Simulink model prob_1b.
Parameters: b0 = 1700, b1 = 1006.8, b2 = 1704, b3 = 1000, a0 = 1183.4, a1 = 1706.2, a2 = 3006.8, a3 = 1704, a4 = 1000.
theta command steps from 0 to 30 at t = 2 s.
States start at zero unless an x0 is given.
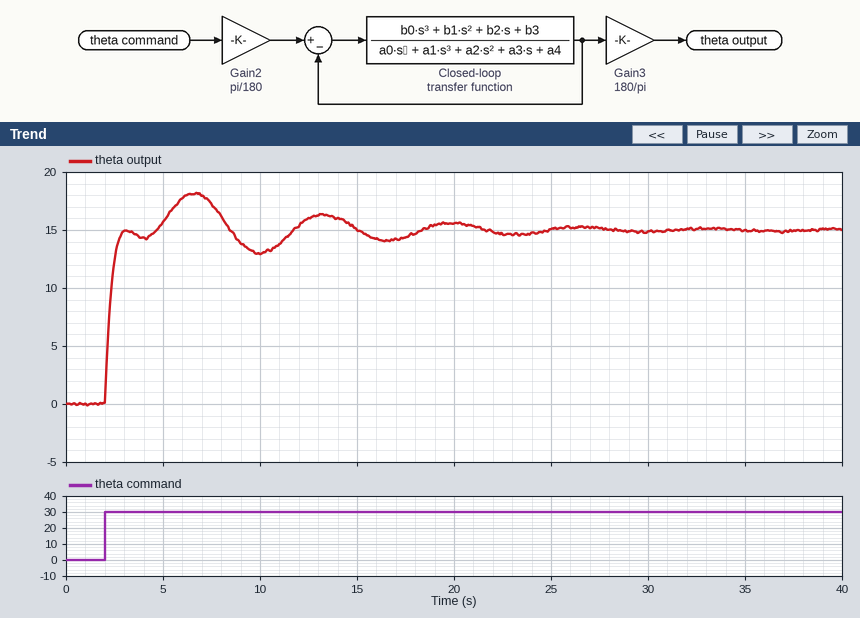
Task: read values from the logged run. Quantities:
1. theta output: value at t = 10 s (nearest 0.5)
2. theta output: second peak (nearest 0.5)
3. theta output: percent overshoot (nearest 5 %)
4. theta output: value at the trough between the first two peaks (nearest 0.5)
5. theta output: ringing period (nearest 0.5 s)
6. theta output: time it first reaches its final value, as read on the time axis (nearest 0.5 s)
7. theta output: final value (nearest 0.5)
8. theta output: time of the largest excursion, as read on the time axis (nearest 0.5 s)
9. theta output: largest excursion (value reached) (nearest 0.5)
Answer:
13.0
16.5
20 %
13.0
6.5 s
4.5 s
15.0
6.5 s
18.0
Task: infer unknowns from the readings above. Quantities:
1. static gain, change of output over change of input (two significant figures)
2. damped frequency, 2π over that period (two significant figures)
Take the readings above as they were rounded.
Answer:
0.50
0.97 rad/s
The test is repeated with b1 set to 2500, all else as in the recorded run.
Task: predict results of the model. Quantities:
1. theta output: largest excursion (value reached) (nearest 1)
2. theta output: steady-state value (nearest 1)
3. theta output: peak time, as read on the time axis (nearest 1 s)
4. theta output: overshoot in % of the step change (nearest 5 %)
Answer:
19
15
3 s
25 %
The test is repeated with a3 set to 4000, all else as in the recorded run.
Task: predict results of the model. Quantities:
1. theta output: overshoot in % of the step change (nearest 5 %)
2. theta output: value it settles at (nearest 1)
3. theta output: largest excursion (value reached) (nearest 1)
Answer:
25 %
15
19
